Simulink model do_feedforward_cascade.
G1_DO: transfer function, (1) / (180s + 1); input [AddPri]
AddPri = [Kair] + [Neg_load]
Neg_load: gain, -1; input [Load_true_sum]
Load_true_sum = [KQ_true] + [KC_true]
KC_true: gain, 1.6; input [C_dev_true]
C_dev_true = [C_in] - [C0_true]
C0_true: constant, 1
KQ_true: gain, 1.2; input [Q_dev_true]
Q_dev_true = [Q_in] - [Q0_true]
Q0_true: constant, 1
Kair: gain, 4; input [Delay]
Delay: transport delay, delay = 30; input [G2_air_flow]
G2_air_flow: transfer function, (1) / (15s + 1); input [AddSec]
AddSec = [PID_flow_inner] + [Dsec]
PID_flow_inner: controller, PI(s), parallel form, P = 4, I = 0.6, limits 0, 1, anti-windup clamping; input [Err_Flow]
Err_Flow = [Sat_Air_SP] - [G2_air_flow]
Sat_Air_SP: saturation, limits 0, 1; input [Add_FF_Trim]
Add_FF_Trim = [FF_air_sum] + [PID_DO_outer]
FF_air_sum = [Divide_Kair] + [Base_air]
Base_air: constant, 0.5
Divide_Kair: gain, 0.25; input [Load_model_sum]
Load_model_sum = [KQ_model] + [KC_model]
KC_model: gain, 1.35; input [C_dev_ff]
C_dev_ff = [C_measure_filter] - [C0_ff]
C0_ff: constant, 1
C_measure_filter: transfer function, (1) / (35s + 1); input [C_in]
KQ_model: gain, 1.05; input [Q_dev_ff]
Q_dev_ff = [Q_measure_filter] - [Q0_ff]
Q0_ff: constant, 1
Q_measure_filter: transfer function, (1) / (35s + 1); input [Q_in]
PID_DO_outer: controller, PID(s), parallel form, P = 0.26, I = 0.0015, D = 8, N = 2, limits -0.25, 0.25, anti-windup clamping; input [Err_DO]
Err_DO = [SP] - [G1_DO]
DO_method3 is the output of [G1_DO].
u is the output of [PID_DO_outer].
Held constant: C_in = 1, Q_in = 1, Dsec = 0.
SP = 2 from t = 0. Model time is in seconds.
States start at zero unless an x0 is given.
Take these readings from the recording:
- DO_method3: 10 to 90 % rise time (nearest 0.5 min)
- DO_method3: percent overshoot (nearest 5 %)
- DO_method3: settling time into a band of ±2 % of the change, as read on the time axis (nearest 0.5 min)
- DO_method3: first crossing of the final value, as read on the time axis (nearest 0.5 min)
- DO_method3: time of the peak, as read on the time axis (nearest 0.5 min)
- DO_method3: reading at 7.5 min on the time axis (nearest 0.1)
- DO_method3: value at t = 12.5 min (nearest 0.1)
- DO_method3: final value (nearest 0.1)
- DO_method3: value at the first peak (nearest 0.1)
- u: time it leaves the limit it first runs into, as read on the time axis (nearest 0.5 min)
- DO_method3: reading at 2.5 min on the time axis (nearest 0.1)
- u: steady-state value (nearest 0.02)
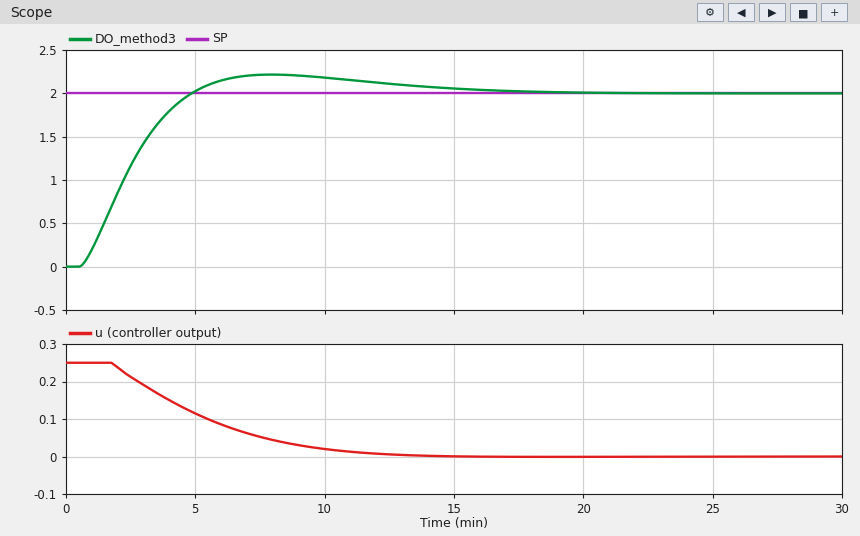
3.0 min
10 %
16.0 min
5.0 min
8.0 min
2.2
2.1
2.0
2.2
2.0 min
1.2
0.00
